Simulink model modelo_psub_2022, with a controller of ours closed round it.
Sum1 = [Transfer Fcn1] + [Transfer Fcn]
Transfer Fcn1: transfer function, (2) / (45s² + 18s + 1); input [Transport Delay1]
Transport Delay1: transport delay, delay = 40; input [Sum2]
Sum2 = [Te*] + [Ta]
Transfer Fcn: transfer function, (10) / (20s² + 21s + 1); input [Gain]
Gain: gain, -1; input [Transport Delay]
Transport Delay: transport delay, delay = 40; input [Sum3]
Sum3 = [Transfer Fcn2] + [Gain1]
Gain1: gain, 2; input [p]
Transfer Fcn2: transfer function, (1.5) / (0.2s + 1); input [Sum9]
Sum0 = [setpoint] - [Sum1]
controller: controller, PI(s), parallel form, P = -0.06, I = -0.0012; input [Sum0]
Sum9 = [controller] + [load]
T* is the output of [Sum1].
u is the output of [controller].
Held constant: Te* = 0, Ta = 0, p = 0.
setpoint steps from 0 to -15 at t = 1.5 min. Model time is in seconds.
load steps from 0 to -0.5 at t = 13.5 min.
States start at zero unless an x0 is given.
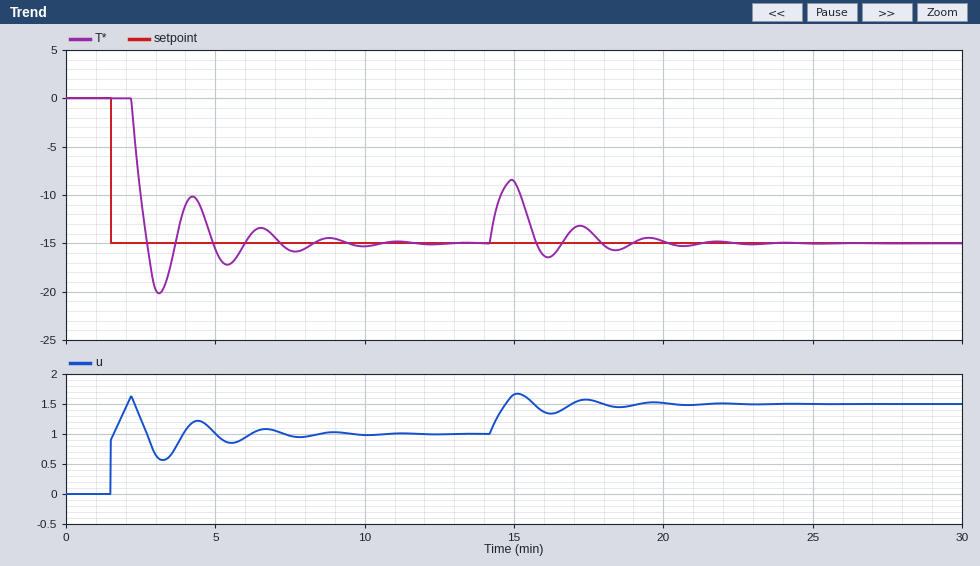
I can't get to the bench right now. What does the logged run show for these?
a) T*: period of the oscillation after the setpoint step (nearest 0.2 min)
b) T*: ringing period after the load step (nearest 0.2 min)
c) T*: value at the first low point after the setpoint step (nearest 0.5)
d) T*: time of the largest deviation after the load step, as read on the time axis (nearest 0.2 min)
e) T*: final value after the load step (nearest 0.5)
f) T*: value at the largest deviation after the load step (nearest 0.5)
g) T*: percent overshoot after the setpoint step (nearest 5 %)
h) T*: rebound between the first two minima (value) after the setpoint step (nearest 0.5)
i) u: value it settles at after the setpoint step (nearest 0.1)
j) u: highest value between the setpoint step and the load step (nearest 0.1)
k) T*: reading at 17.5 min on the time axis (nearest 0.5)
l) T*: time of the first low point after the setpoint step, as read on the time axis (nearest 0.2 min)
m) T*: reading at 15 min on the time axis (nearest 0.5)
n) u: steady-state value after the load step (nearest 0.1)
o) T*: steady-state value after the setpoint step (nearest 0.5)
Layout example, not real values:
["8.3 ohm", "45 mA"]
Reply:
["2.2 min", "2.2 min", "-20.0", "15.0 min", "-15.0", "-8.5", "35 %", "-10.0", "1.0", "1.6", "-13.5", "3.2 min", "-8.5", "1.5", "-15.0"]
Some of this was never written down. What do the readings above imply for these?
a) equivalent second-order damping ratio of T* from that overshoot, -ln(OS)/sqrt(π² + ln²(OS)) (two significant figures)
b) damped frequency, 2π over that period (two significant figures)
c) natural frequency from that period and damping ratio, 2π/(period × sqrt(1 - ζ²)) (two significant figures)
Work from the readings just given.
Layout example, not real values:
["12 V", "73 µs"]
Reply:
["0.32", "2.9 rad/min", "3.0 rad/min"]
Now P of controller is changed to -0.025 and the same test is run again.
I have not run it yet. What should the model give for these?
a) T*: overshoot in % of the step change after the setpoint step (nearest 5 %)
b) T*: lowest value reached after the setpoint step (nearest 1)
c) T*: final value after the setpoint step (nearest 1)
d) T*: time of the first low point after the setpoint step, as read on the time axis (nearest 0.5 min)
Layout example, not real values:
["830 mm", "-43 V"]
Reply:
["25 %", "-19", "-15", "4.0 min"]
